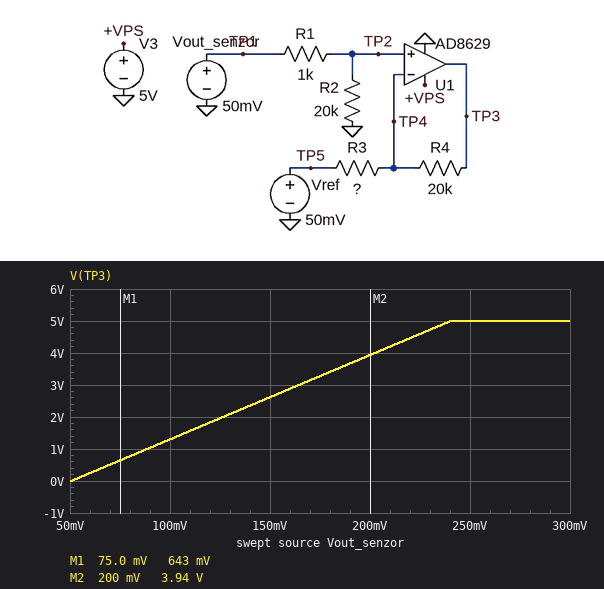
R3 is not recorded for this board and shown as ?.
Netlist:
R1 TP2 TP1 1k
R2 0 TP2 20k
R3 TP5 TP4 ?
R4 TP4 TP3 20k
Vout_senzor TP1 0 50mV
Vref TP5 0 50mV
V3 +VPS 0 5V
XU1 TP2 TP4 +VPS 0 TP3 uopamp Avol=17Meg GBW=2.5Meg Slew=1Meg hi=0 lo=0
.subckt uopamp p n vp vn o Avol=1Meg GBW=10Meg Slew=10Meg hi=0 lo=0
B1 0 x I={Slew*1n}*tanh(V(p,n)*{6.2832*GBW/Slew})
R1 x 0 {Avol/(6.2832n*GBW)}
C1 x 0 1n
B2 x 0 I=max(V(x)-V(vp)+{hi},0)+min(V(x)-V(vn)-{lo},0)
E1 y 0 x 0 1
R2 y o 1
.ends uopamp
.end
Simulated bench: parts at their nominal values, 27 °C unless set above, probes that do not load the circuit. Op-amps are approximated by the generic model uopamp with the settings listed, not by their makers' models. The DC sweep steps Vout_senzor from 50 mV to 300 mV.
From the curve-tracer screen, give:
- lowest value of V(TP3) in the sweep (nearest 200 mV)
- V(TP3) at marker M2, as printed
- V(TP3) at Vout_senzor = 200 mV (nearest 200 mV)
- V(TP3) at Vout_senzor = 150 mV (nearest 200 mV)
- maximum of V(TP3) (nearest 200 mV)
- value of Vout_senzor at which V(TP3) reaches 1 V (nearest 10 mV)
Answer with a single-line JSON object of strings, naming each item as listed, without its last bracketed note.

{"lowest value of V(TP3) in the sweep": "0 V", "V(TP3) at marker M2, as printed": "3.94 V", "V(TP3) at Vout_senzor = 200 mV": "4.0 V", "V(TP3) at Vout_senzor = 150 mV": "2.6 V", "maximum of V(TP3)": "5.0 V", "value of Vout_senzor at which V(TP3) reaches 1 V": "90 mV"}
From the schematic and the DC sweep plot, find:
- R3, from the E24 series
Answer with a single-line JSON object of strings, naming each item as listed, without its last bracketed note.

{"R3, from the E24 series": "750 Ω"}
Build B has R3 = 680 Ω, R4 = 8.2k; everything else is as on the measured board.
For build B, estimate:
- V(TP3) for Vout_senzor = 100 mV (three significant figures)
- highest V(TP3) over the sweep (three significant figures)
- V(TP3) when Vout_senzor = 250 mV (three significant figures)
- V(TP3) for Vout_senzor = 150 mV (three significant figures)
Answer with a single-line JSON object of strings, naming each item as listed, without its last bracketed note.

{"V(TP3) for Vout_senzor = 100 mV": "641 mV", "highest V(TP3) over the sweep": "3.13 V", "V(TP3) when Vout_senzor = 250 mV": "2.51 V", "V(TP3) for Vout_senzor = 150 mV": "1.26 V"}
